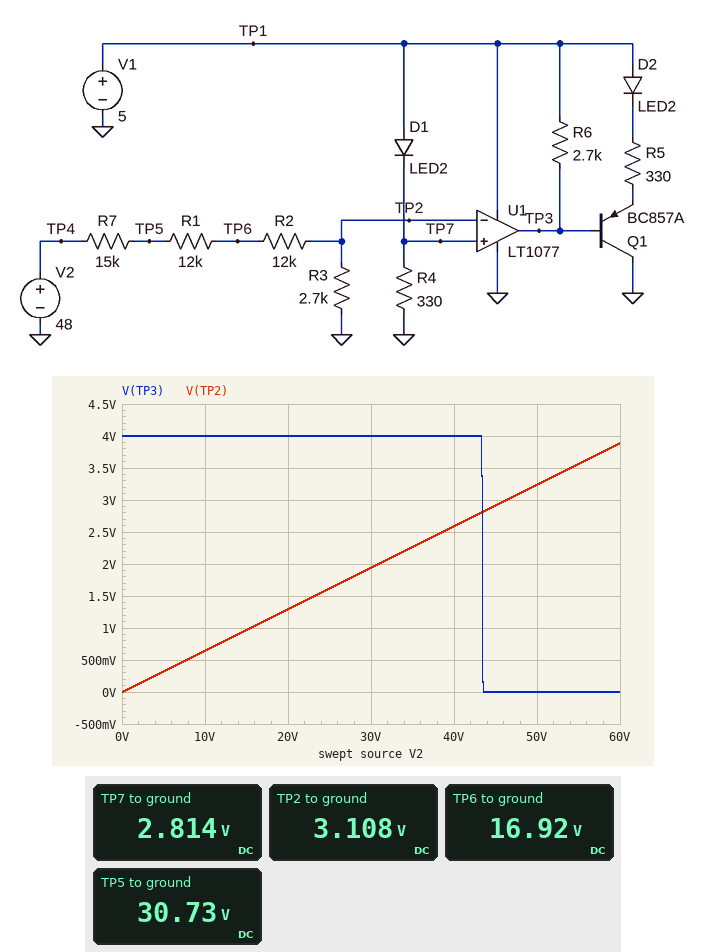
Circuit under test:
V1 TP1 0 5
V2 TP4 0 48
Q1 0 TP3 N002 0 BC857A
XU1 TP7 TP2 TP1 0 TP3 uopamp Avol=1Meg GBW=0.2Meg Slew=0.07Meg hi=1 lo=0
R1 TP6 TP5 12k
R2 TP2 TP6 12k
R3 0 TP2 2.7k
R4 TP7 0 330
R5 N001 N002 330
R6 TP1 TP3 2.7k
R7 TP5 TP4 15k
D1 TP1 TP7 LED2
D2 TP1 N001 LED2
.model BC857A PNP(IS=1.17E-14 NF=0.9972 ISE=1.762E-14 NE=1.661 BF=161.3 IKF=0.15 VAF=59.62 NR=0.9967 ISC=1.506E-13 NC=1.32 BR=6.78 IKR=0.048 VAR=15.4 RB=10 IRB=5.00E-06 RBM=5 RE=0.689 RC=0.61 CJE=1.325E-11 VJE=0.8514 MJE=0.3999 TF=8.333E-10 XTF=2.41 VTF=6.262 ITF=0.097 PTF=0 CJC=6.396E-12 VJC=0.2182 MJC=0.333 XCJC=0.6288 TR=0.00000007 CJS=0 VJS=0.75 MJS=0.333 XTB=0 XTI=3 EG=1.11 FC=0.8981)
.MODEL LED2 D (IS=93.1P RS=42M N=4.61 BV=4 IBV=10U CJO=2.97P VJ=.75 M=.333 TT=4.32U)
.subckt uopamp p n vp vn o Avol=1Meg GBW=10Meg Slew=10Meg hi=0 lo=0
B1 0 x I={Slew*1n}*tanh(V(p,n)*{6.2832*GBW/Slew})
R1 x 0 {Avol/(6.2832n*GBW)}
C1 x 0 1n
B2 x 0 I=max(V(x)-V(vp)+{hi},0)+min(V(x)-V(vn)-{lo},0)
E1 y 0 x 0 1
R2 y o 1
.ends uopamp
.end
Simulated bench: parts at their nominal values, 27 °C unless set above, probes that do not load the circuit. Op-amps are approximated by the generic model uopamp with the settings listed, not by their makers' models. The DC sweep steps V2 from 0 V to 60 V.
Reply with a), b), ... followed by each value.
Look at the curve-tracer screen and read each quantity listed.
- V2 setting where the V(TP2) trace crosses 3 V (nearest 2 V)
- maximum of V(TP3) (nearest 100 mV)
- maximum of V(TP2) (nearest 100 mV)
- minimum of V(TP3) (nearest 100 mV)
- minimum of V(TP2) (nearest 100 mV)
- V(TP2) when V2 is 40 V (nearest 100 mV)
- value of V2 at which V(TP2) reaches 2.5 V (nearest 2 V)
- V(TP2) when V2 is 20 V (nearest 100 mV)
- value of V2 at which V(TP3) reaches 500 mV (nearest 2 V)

a) 46 V
b) 4.0 V
c) 3.9 V
d) 0 V
e) 0 V
f) 2.6 V
g) 38 V
h) 1.3 V
i) 44 V
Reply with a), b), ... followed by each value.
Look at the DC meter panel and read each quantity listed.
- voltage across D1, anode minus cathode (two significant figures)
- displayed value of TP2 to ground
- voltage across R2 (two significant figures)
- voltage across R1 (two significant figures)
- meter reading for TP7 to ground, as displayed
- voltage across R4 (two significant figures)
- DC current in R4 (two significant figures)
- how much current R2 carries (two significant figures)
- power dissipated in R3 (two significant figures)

a) 2.2 V
b) 3.108 V
c) 14 V
d) 14 V
e) 2.814 V
f) 2.8 V
g) 8.5 mA
h) 1.2 mA
i) 3.6 mW
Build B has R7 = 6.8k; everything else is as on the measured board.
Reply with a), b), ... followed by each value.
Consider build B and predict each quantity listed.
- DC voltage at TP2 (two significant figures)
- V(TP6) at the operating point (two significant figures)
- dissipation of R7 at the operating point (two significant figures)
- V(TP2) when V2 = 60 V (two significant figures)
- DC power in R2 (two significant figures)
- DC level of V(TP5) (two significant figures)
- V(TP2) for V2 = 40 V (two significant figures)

a) 3.9 V
b) 21 V
c) 14 mW
d) 4.8 V
e) 25 mW
f) 38 V
g) 3.2 V
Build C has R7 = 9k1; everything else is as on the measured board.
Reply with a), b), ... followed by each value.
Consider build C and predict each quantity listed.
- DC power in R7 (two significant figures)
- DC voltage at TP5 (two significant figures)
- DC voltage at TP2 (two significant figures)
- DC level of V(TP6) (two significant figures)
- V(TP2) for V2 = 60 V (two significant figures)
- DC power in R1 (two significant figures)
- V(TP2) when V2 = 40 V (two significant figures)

a) 16 mW
b) 36 V
c) 3.6 V
d) 20 V
e) 4.5 V
f) 22 mW
g) 3.0 V
